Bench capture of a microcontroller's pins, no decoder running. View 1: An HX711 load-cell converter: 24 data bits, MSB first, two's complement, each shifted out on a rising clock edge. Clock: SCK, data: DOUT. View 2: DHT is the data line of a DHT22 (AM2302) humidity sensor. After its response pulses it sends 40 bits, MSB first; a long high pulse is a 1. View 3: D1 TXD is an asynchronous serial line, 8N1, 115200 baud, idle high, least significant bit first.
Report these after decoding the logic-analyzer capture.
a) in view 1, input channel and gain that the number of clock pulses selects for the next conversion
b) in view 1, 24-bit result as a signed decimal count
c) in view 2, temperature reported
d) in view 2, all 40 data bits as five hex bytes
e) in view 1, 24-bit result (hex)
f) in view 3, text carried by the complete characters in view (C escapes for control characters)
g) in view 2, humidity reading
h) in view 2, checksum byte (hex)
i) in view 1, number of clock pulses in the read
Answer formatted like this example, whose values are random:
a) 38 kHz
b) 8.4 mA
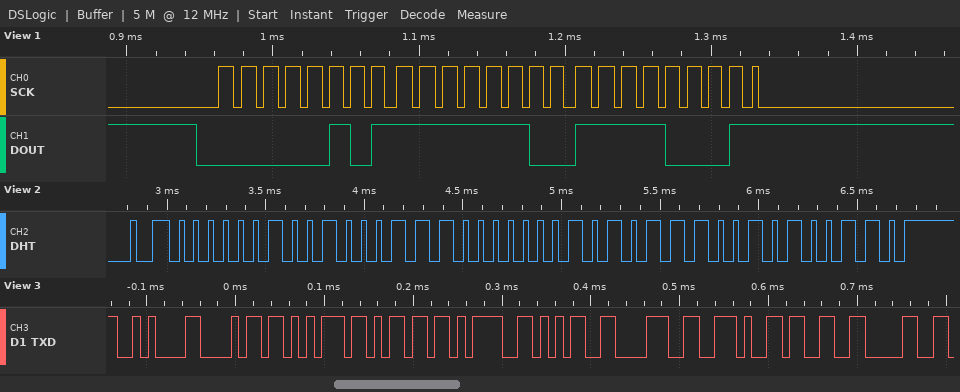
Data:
a) channel A, gain 128
b) 392433
c) 34.8 °C
d) 02 47 01 5C A6
e) 0x05FCF1
f) "\nhum=58.30"
g) 58.3 %
h) 0xA6
i) 25
